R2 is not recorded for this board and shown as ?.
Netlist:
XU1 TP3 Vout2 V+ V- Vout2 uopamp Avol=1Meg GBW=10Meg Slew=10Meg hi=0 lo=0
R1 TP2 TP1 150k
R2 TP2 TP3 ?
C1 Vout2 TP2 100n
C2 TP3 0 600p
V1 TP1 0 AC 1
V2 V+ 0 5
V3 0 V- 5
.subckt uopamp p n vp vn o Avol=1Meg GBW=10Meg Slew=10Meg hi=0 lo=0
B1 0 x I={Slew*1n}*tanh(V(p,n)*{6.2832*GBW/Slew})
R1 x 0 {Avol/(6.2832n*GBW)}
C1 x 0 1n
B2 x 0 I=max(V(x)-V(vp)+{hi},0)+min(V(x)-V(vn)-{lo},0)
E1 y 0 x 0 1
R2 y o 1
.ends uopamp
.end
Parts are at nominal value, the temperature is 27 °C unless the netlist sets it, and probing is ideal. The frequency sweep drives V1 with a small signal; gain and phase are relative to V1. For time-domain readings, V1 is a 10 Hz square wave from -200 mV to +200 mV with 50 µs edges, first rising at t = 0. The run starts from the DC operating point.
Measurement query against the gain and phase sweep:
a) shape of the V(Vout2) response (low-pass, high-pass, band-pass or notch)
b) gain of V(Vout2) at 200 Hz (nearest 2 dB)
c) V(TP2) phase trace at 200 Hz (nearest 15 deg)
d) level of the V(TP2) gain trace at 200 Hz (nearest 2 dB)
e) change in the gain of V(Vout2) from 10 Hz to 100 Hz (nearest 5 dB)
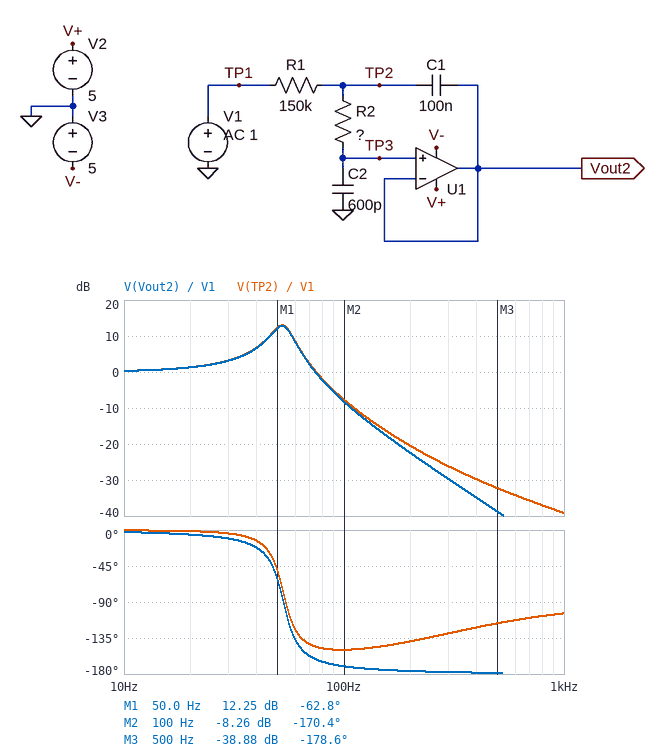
low-pass
-22 dB
-135 deg
-20 dB
-10 dB
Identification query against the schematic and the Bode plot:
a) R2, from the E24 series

1 MΩ
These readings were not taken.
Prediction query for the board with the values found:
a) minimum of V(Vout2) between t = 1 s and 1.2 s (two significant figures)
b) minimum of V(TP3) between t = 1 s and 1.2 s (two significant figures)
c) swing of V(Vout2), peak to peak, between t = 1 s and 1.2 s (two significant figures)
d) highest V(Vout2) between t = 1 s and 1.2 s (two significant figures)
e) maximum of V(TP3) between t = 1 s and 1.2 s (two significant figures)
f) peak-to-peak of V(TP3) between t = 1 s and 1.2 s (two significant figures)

-510 mV
-510 mV
1.0 V
510 mV
510 mV
1.0 V
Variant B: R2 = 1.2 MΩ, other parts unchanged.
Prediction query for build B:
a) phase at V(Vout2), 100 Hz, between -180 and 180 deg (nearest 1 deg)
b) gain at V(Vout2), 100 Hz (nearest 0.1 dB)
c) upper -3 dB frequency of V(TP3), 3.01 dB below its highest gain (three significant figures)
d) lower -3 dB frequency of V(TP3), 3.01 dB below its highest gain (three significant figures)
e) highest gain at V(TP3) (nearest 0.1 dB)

-171 deg
-10.4 dB
53.4 Hz
41.2 Hz
12.2 dB
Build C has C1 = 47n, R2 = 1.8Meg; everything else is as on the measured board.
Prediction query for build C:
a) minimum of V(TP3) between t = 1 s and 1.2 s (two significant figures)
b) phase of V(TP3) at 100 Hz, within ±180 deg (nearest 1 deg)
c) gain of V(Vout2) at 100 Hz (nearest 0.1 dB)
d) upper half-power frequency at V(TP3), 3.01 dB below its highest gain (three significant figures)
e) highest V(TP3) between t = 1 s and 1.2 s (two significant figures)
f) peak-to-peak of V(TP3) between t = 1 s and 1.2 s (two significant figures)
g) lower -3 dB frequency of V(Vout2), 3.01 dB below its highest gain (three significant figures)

-400 mV
-160 deg
-6.6 dB
66.4 Hz
400 mV
800 mV
40.6 Hz
